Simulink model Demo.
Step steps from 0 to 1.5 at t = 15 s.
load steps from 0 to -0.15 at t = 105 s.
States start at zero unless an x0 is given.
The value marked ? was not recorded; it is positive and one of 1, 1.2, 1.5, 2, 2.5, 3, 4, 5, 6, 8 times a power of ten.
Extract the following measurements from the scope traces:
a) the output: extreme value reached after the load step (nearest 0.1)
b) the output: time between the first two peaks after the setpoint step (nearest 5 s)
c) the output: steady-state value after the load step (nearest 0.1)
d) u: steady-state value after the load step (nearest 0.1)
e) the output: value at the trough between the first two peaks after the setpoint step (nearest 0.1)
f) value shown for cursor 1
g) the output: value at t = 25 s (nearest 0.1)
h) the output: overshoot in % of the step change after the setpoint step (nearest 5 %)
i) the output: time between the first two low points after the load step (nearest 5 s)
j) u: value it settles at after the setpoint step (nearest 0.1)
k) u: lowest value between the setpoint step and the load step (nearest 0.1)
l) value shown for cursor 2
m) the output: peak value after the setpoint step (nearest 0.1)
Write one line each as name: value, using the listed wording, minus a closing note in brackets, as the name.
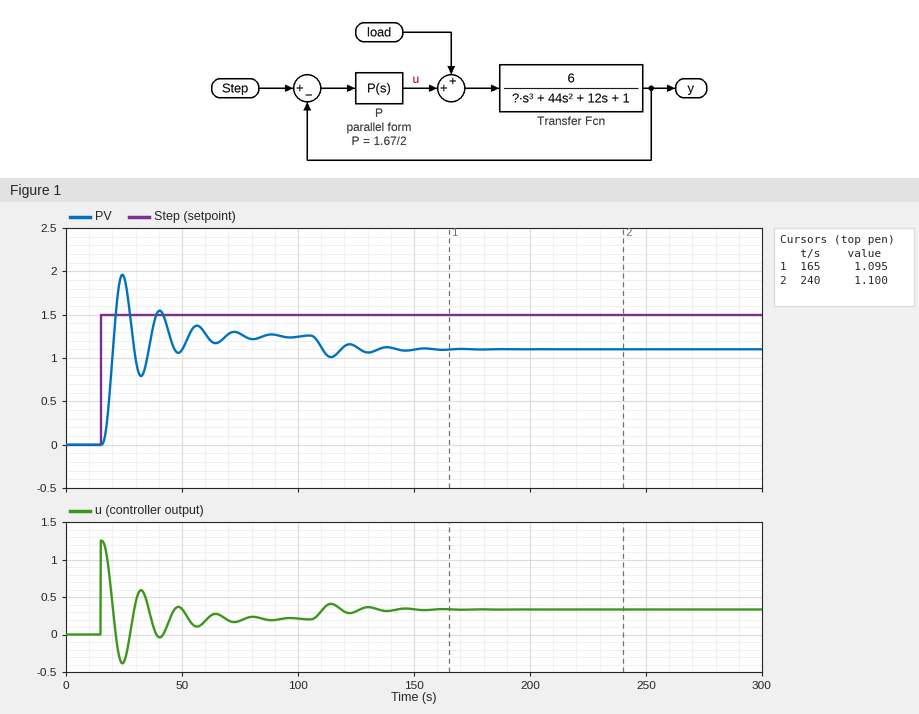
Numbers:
the output: extreme value reached after the load step: 1.0
the output: time between the first two peaks after the setpoint step: 15 s
the output: steady-state value after the load step: 1.1
u: steady-state value after the load step: 0.3
the output: value at the trough between the first two peaks after the setpoint step: 0.8
value shown for cursor 1: 1.095
the output: value at t = 25 s: 1.9
the output: overshoot in % of the step change after the setpoint step: 55 %
the output: time between the first two low points after the load step: 15 s
u: value it settles at after the setpoint step: 0.2
u: lowest value between the setpoint step and the load step: -0.4
value shown for cursor 2: 1.100
the output: peak value after the setpoint step: 2.0
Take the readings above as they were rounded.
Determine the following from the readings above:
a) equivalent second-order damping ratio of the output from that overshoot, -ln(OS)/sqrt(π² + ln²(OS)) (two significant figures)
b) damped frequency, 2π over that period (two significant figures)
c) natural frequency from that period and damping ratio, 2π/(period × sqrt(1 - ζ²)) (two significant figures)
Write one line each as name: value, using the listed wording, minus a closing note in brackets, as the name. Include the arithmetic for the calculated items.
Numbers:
equivalent second-order damping ratio of the output from that overshoot, -ln(OS)/sqrt(π² + ln²(OS)): ln(0.55) = -0.598; 0.598 / sqrt(9.870 + 0.357) = 0.19
damped frequency, 2π over that period: 2π / 15 = 0.42 rad/s
natural frequency from that period and damping ratio, 2π/(period × sqrt(1 - ζ²)): 2π / (15 × sqrt(1 - 0.19²)) = 0.43 rad/s
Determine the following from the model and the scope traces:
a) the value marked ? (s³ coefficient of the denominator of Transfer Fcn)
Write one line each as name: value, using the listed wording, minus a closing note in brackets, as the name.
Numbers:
the value marked ?: 50
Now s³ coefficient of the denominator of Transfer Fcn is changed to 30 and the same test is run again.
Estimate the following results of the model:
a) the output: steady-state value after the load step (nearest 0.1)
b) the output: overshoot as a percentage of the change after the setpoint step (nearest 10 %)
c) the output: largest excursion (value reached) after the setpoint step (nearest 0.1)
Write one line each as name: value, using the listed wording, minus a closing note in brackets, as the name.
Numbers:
the output: steady-state value after the load step: 1.1
the output: overshoot as a percentage of the change after the setpoint step: 40 %
the output: largest excursion (value reached) after the setpoint step: 1.8
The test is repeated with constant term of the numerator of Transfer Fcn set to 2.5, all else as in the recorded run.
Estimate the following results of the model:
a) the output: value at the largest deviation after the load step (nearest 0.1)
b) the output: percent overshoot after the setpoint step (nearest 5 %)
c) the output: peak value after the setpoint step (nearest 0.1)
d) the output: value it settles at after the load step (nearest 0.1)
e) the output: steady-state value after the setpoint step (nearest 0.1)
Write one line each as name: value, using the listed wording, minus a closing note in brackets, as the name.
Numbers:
the output: value at the largest deviation after the load step: 0.9
the output: percent overshoot after the setpoint step: 25 %
the output: peak value after the setpoint step: 1.3
the output: value it settles at after the load step: 0.9
the output: steady-state value after the setpoint step: 1.0
